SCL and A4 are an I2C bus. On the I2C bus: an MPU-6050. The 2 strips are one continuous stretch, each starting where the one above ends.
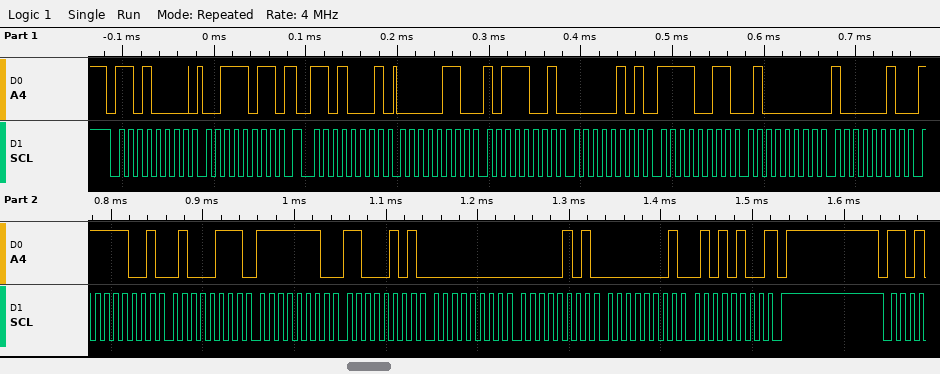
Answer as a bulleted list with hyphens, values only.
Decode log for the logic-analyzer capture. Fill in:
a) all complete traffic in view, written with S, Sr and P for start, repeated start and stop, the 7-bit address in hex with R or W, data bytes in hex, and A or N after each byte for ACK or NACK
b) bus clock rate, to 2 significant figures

- S 68W A 3B A Sr 68R A 06 A B9 A 05 A F3 A 40 A 82 A F9 A 47 A FE A C5 A 00 A 05 A 01 A 54 N P
- 100 kHz
